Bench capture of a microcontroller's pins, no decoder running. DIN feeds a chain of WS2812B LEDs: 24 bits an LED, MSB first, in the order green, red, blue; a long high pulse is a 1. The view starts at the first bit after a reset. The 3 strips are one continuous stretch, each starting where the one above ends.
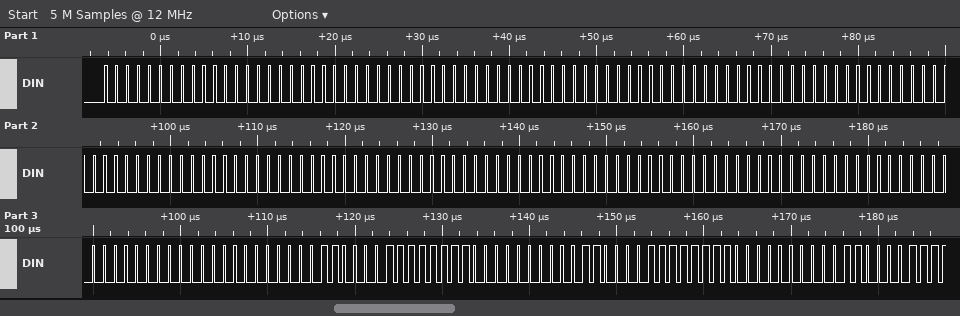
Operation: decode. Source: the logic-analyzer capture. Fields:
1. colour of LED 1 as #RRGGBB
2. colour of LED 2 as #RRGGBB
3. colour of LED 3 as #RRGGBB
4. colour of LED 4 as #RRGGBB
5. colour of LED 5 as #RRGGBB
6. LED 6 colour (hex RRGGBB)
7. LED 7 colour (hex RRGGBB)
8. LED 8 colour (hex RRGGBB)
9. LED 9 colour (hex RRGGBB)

#000000
#000000
#000000
#000000
#000000
#000000
#000000
#3000FF
#3000FF
